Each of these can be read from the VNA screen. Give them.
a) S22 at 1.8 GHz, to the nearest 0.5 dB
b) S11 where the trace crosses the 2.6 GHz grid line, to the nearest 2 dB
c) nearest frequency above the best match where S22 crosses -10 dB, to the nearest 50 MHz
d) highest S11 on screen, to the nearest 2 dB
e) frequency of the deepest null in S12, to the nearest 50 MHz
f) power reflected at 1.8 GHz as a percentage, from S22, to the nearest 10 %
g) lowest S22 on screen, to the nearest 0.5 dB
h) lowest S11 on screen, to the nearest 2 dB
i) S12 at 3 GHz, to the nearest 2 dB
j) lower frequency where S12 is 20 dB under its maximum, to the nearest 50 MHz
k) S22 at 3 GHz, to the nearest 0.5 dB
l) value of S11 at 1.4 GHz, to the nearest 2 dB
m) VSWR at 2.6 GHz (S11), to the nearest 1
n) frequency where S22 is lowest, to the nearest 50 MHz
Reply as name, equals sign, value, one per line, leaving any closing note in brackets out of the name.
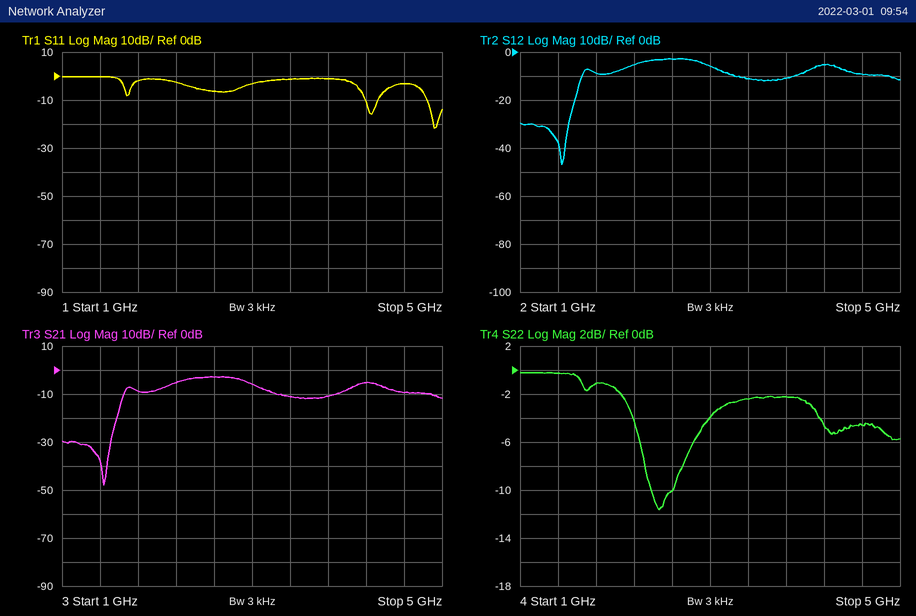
S22 at 1.8 GHz, to the nearest 0.5 dB = -1.0 dB
S11 where the trace crosses the 2.6 GHz grid line, to the nearest 2 dB = -6 dB
nearest frequency above the best match where S22 crosses -10 dB, to the nearest 50 MHz = 2.60 GHz
highest S11 on screen, to the nearest 2 dB = 0 dB
frequency of the deepest null in S12, to the nearest 50 MHz = 1.45 GHz
power reflected at 1.8 GHz as a percentage, from S22, to the nearest 10 % = 80 %
lowest S22 on screen, to the nearest 0.5 dB = -11.5 dB
lowest S11 on screen, to the nearest 2 dB = -22 dB
S12 at 3 GHz, to the nearest 2 dB = -6 dB
lower frequency where S12 is 20 dB under its maximum, to the nearest 50 MHz = 1.55 GHz
S22 at 3 GHz, to the nearest 0.5 dB = -4.0 dB
value of S11 at 1.4 GHz, to the nearest 2 dB = 0 dB
VSWR at 2.6 GHz (S11), to the nearest 1 = 3
frequency where S22 is lowest, to the nearest 50 MHz = 2.45 GHz
